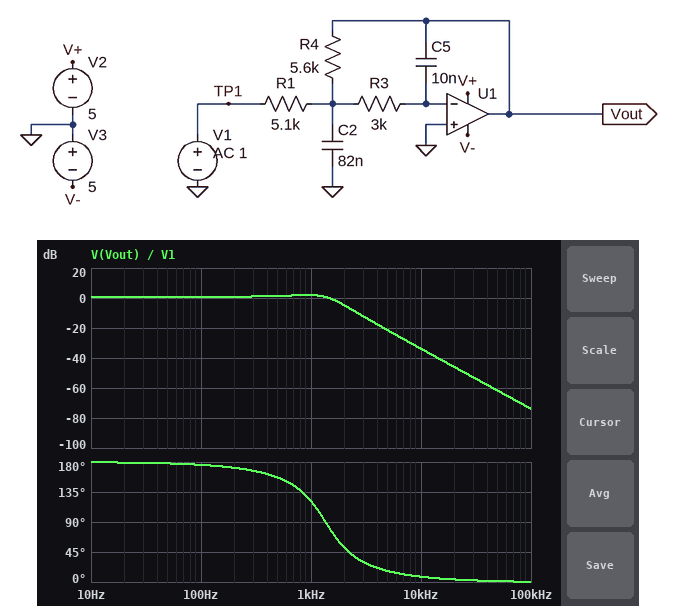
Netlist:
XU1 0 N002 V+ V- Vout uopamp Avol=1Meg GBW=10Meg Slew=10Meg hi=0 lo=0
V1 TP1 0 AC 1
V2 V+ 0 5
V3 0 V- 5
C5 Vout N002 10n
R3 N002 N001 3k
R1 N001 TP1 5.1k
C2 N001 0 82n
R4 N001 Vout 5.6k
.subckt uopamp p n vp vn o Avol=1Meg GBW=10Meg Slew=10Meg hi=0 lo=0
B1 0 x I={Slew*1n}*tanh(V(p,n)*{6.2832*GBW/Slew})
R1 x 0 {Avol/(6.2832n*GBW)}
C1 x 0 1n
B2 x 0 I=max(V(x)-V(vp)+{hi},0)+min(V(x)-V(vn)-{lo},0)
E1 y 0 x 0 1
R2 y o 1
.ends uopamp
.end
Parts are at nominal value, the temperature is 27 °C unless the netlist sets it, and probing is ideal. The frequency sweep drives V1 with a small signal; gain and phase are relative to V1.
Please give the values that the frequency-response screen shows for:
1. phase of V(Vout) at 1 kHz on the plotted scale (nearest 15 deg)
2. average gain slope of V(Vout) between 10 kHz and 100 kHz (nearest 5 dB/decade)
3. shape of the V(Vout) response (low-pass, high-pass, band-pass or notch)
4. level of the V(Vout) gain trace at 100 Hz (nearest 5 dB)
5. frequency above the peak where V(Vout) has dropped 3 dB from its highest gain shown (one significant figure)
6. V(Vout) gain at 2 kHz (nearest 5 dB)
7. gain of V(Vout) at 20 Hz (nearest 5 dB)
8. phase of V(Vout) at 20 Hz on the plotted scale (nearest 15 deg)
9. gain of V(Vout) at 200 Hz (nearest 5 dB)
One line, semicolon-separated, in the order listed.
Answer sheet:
120 deg; -40 dB/decade; low-pass; 0 dB; 2 kHz; -5 dB; 0 dB; 180 deg; 0 dB
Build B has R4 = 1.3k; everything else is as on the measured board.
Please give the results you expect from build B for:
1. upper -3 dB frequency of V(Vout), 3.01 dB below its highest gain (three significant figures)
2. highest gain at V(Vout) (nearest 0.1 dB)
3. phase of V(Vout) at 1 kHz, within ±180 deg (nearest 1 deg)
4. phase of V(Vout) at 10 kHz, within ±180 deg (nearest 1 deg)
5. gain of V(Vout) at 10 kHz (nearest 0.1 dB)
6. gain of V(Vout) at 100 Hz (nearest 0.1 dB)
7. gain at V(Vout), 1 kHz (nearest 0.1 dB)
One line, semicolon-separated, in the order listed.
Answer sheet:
3.33 kHz; -9.9 dB; 160 deg; 15 deg; -33.5 dB; -11.9 dB; -11.2 dB
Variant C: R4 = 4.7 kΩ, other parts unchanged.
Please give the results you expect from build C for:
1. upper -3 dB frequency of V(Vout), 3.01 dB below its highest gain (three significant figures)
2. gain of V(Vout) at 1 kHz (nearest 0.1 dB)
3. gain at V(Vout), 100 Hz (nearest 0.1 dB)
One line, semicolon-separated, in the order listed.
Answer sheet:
1.74 kHz; 0.7 dB; -0.7 dB
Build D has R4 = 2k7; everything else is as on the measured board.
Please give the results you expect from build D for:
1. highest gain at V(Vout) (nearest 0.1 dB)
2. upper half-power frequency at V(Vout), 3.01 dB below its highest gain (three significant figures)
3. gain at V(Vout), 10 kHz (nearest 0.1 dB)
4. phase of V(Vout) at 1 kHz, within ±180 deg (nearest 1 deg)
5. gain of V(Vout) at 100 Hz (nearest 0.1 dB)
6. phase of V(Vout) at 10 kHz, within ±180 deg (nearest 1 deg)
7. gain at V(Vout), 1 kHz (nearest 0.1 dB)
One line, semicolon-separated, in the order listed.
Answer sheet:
-3.6 dB; 2.31 kHz; -33.7 dB; 148 deg; -5.5 dB; 10 deg; -4.3 dB
